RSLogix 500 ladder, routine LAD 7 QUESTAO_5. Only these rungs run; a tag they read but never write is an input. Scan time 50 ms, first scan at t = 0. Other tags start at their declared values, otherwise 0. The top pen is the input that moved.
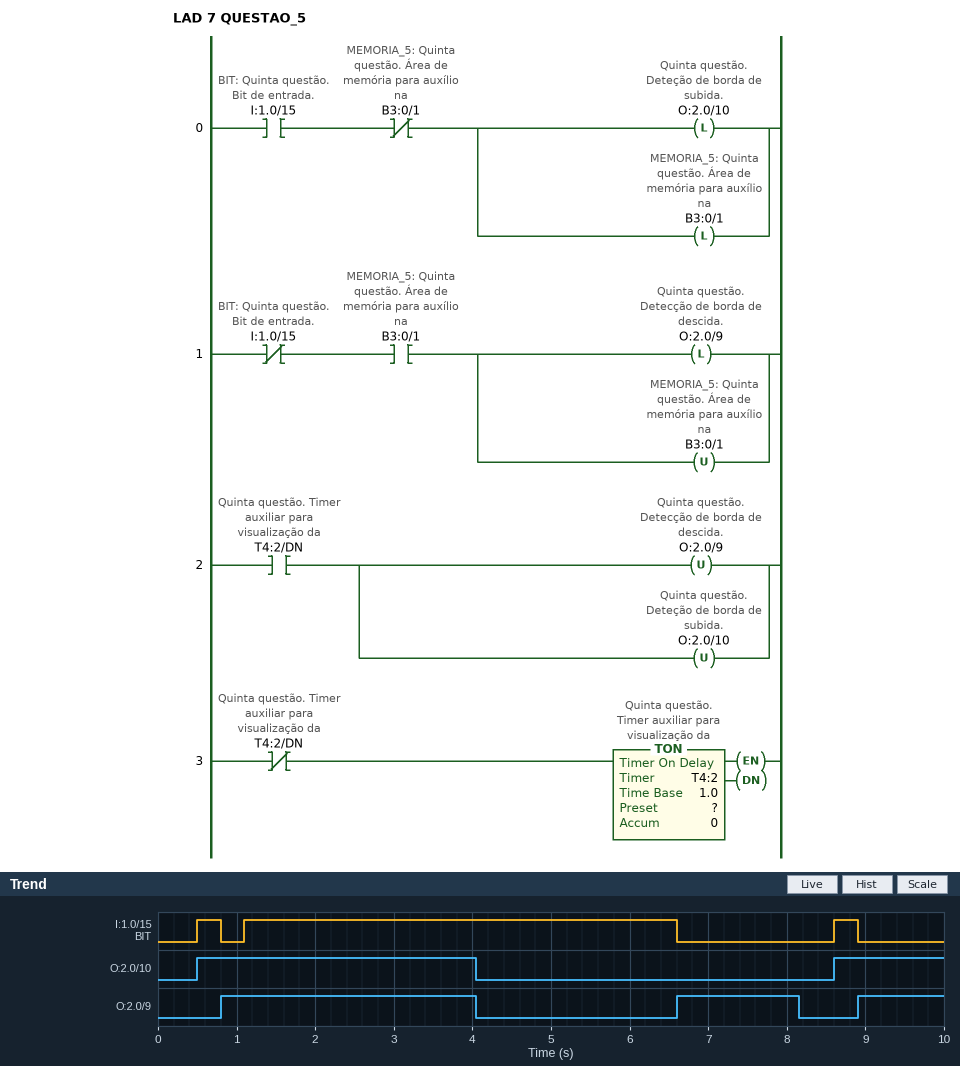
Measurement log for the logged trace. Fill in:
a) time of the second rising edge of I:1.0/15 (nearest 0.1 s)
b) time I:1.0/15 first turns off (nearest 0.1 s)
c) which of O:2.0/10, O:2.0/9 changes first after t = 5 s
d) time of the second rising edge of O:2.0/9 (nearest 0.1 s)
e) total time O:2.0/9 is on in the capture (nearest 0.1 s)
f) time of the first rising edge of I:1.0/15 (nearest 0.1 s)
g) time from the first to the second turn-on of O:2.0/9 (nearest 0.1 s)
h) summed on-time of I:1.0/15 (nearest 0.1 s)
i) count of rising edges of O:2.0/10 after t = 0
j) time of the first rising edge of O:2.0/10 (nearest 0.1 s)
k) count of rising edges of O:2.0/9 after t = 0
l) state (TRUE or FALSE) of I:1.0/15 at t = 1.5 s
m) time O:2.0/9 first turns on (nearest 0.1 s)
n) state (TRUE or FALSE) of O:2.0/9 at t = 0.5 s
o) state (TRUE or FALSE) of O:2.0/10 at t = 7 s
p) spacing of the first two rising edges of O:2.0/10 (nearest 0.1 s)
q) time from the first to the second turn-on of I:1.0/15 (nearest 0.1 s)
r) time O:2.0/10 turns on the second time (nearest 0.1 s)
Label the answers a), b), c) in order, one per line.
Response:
a) 1.1 s
b) 0.8 s
c) O:2.0/9
d) 6.6 s
e) 5.9 s
f) 0.5 s
g) 5.8 s
h) 6.1 s
i) 2
j) 0.5 s
k) 3
l) TRUE
m) 0.8 s
n) FALSE
o) FALSE
p) 8.1 s
q) 0.6 s
r) 8.6 s
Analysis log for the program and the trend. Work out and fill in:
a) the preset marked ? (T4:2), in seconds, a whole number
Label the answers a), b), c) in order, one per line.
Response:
a) 4 s
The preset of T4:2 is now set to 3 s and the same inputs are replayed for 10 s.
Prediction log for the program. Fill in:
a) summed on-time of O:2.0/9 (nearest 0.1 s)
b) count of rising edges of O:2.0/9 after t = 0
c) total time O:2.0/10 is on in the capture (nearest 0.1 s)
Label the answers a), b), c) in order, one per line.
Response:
a) 4.9 s
b) 2
c) 3.2 s
